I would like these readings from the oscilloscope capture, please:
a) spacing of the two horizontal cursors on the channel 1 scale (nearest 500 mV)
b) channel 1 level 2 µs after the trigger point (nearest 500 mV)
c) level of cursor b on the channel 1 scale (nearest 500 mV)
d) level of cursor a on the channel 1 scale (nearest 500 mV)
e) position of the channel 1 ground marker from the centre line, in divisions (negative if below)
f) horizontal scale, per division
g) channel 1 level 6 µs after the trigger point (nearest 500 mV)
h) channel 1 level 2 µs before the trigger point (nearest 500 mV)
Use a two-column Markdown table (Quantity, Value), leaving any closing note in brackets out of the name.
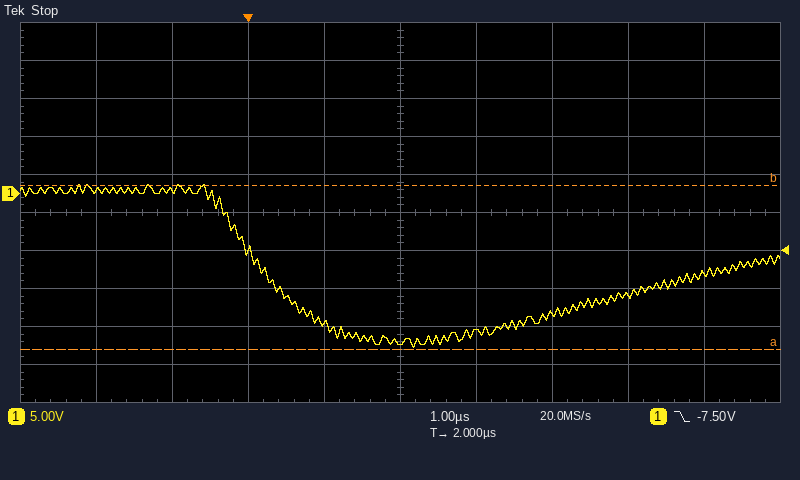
| Quantity | Value |
|---|---|
| spacing of the two horizontal cursors on the channel 1 scale | 21.5 V |
| channel 1 level 2 µs after the trigger point | -19.5 V |
| level of cursor b on the channel 1 scale | 1.0 V |
| level of cursor a on the channel 1 scale | -20.5 V |
| position of the channel 1 ground marker from the centre line, in divisions | +0.5 div |
| horizontal scale, per division | 1 µs |
| channel 1 level 6 µs after the trigger point | -10.5 V |
| channel 1 level 2 µs before the trigger point | 500 mV |
